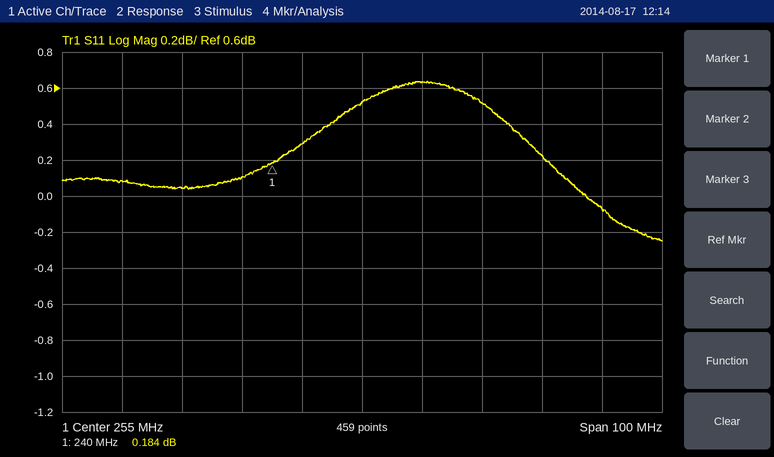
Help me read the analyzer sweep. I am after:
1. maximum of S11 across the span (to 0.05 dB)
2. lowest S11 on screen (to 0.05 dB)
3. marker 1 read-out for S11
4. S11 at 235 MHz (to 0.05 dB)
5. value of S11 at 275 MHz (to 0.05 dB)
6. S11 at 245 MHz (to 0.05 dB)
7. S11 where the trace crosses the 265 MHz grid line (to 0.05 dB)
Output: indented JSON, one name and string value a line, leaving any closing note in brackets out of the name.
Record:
{
  "maximum of S11 across the span": "0.65 dB",
  "lowest S11 on screen": "-0.25 dB",
  "marker 1 read-out for S11": "0.184 dB",
  "S11 at 235 MHz": "0.10 dB",
  "value of S11 at 275 MHz": "0.50 dB",
  "S11 at 245 MHz": "0.30 dB",
  "S11 where the trace crosses the 265 MHz grid line": "0.65 dB"
}
